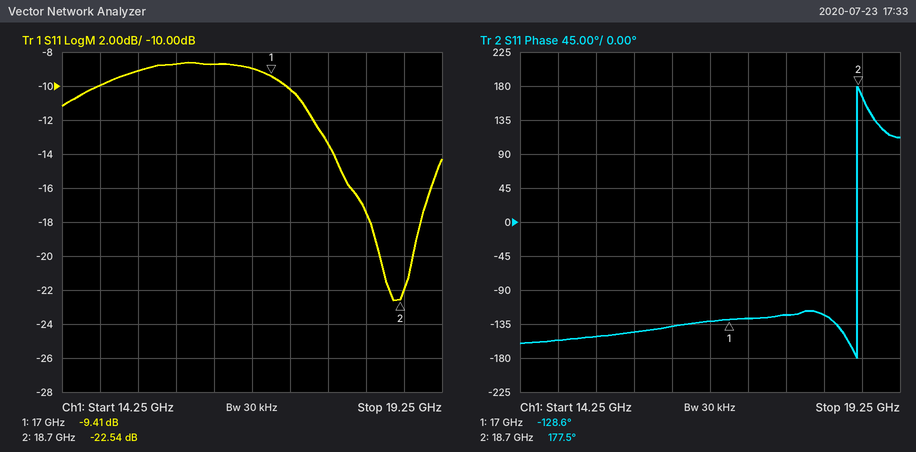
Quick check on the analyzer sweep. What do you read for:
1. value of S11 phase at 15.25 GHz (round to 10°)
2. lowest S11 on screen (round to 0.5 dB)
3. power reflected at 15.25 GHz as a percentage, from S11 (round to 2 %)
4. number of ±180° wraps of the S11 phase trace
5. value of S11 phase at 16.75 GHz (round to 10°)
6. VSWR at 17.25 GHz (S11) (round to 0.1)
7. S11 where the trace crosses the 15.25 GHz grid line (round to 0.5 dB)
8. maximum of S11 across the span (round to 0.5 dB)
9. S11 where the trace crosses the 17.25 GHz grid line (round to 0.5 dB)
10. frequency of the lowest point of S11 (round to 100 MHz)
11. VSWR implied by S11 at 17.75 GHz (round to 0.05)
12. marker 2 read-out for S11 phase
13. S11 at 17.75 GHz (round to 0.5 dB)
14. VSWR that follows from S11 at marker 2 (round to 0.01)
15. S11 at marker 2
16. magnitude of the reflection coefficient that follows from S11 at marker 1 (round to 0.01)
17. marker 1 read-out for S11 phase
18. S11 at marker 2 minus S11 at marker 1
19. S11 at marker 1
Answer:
-150°
-22.5 dB
12 %
1
-130°
1.9
-9.0 dB
-8.5 dB
-10.0 dB
18.6 GHz
1.55
177.5°
-13.5 dB
1.16
-22.54 dB
0.34
-128.6°
-13.13 dB
-9.41 dB
